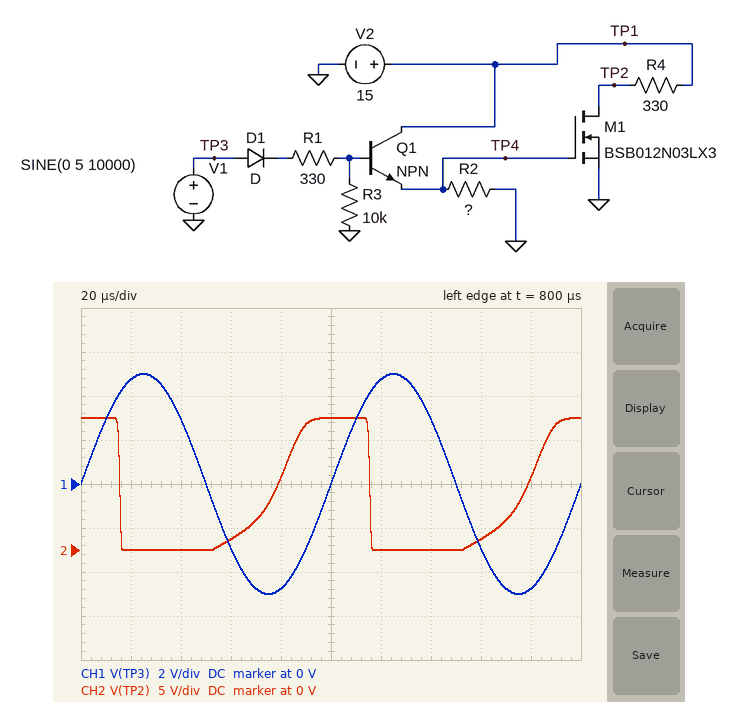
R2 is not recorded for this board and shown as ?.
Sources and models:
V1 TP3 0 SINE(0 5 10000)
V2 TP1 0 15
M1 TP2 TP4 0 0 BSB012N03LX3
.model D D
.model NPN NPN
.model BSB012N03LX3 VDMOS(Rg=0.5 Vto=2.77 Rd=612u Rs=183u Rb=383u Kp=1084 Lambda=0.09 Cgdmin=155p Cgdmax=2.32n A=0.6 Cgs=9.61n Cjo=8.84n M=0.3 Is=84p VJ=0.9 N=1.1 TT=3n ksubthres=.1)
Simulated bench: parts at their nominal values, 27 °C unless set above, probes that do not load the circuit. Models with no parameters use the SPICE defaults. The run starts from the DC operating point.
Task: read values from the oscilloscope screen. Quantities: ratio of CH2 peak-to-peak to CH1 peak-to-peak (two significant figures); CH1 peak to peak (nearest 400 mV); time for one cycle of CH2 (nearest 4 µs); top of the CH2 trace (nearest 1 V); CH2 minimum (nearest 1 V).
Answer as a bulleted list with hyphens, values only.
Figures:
- 1.5
- 10.0 V
- 100 µs
- 15 V
- 0 V
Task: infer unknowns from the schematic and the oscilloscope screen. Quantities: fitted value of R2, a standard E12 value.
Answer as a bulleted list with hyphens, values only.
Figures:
- 6.8 kΩ
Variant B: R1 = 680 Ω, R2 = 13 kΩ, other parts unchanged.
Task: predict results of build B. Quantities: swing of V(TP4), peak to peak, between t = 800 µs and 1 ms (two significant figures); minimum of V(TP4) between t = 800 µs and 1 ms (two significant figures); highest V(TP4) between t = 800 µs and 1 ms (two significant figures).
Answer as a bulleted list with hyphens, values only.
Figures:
- 860 mV
- 2.5 V
- 3.3 V
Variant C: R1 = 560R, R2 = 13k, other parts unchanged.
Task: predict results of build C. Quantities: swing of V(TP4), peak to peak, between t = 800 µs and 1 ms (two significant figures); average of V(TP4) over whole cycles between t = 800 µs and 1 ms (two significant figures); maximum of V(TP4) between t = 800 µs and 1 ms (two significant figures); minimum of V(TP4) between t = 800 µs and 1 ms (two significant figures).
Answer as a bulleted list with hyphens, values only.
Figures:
- 900 mV
- 2.8 V
- 3.4 V
- 2.5 V
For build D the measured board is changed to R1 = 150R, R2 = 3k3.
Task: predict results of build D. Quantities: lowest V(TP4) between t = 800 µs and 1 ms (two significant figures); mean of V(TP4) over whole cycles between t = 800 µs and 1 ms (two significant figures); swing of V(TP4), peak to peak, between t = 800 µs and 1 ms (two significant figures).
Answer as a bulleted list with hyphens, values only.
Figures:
- 540 mV
- 2.0 V
- 3.0 V
